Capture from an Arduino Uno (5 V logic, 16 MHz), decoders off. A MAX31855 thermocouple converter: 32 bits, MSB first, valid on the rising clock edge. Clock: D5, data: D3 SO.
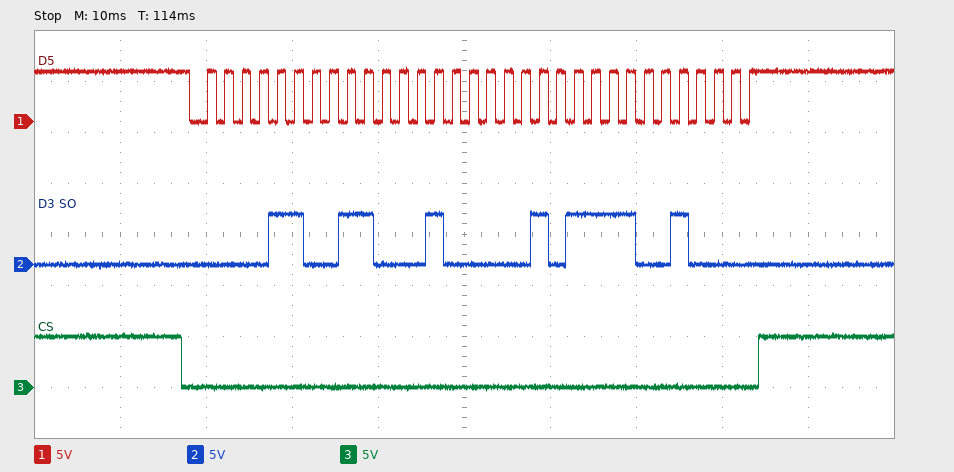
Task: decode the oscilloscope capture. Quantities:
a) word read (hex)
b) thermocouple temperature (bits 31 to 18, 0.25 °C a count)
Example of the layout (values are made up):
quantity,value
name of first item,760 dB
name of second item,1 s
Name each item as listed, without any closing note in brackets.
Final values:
quantity,value
word read,0x0CC41790
thermocouple temperature,204.25 °C
